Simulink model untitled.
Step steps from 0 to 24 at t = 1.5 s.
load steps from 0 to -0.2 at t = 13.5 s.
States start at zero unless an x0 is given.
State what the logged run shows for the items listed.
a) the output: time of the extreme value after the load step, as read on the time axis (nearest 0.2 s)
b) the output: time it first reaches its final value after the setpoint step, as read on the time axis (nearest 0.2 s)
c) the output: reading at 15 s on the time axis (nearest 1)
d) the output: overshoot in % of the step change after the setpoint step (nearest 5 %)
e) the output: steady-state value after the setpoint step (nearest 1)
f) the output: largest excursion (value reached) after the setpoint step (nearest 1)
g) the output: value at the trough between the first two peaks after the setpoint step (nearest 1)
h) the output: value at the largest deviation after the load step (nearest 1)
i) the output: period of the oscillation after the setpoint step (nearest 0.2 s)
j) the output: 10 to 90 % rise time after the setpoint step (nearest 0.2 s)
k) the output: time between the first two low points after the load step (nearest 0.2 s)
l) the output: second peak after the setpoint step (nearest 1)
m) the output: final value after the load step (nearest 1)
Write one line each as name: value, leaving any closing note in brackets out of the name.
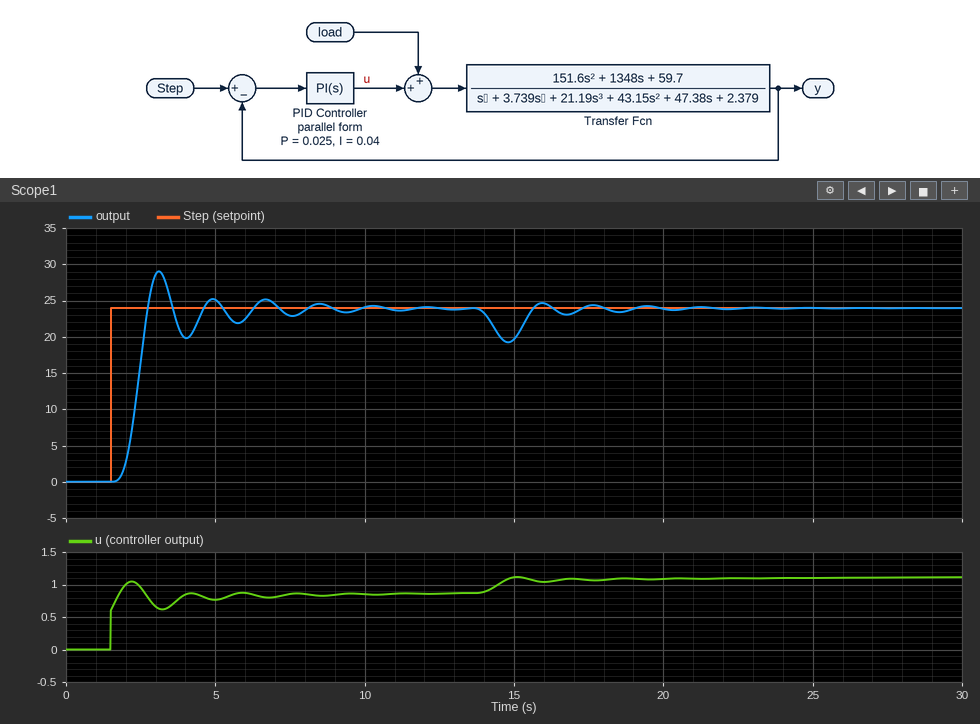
the output: time of the extreme value after the load step, as read on the time axis: 14.8 s
the output: time it first reaches its final value after the setpoint step, as read on the time axis: 2.8 s
the output: reading at 15 s on the time axis: 20
the output: overshoot in % of the step change after the setpoint step: 20 %
the output: steady-state value after the setpoint step: 24
the output: largest excursion (value reached) after the setpoint step: 29
the output: value at the trough between the first two peaks after the setpoint step: 20
the output: value at the largest deviation after the load step: 19
the output: period of the oscillation after the setpoint step: 1.8 s
the output: 10 to 90 % rise time after the setpoint step: 0.6 s
the output: time between the first two low points after the load step: 2.0 s
the output: second peak after the setpoint step: 25
the output: final value after the load step: 24
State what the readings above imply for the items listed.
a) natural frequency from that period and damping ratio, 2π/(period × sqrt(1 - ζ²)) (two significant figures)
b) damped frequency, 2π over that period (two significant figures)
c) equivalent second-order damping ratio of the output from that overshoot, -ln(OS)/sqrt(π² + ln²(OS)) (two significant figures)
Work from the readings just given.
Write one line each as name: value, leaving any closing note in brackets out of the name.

natural frequency from that period and damping ratio, 2π/(period × sqrt(1 - ζ²)): 3.9 rad/s
damped frequency, 2π over that period: 3.5 rad/s
equivalent second-order damping ratio of the output from that overshoot, -ln(OS)/sqrt(π² + ln²(OS)): 0.46
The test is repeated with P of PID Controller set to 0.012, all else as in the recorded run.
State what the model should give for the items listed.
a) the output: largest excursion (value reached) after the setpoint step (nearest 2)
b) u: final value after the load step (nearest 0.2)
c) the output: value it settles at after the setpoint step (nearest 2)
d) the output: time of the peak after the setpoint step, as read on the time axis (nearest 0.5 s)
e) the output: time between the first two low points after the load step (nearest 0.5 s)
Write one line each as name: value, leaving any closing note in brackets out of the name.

the output: largest excursion (value reached) after the setpoint step: 28
u: final value after the load step: 1.2
the output: value it settles at after the setpoint step: 24
the output: time of the peak after the setpoint step, as read on the time axis: 3.5 s
the output: time between the first two low points after the load step: 3.5 s
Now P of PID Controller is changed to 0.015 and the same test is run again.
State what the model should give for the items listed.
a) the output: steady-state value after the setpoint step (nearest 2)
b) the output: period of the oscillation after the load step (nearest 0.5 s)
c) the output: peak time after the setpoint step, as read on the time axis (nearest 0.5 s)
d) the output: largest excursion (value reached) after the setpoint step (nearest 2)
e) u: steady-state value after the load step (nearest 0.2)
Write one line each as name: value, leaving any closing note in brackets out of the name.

the output: steady-state value after the setpoint step: 24
the output: period of the oscillation after the load step: 3.5 s
the output: peak time after the setpoint step, as read on the time axis: 3.5 s
the output: largest excursion (value reached) after the setpoint step: 28
u: steady-state value after the load step: 1.2
